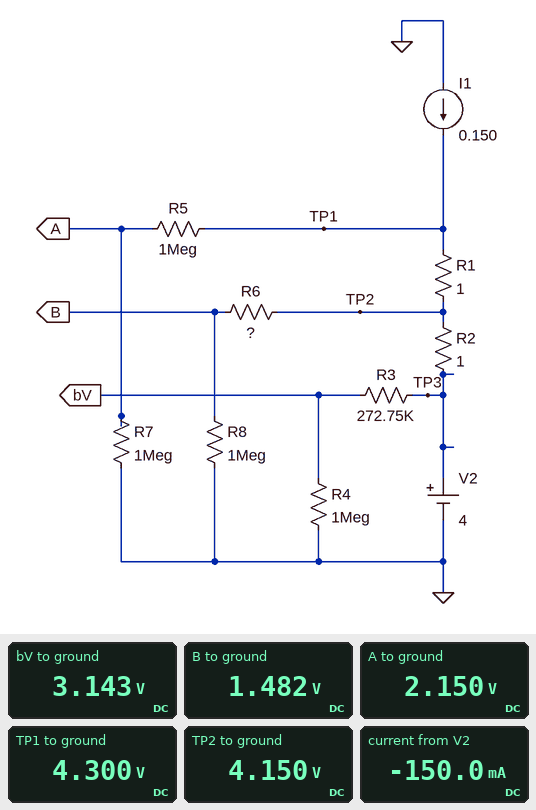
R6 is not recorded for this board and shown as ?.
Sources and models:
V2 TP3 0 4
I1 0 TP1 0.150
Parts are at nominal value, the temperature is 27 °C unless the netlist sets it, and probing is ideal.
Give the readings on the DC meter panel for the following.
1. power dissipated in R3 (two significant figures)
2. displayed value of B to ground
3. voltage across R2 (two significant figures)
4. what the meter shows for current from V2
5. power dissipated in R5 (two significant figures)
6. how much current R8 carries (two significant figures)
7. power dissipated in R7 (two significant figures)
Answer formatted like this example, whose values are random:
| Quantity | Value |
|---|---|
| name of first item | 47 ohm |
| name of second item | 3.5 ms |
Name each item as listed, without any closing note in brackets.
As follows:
| Quantity | Value |
|---|---|
| power dissipated in R3 | 2.7 µW |
| displayed value of B to ground | 1.482 V |
| voltage across R2 | 150 mV |
| what the meter shows for current from V2 | -150.0 mA |
| power dissipated in R5 | 4.6 µW |
| how much current R8 carries | 1.5 µA |
| power dissipated in R7 | 4.6 µW |
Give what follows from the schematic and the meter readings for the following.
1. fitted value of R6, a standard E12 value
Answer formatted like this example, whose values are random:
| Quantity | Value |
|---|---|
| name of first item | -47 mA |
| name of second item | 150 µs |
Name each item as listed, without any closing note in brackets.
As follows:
| Quantity | Value |
|---|---|
| fitted value of R6, a standard E12 value | 1.8 MΩ |
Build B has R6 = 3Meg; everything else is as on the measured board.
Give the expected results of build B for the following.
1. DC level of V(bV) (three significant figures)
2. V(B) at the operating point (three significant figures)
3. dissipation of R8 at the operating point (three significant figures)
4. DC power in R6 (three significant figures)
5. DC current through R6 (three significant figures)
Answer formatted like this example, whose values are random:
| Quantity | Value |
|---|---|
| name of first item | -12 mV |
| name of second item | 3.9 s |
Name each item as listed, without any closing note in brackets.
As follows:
| Quantity | Value |
|---|---|
| DC level of V(bV) | 3.14 V |
| V(B) at the operating point | 1.04 V |
| dissipation of R8 at the operating point | 1.08 µW |
| DC power in R6 | 3.23 µW |
| DC current through R6 | 1.04 µA |
